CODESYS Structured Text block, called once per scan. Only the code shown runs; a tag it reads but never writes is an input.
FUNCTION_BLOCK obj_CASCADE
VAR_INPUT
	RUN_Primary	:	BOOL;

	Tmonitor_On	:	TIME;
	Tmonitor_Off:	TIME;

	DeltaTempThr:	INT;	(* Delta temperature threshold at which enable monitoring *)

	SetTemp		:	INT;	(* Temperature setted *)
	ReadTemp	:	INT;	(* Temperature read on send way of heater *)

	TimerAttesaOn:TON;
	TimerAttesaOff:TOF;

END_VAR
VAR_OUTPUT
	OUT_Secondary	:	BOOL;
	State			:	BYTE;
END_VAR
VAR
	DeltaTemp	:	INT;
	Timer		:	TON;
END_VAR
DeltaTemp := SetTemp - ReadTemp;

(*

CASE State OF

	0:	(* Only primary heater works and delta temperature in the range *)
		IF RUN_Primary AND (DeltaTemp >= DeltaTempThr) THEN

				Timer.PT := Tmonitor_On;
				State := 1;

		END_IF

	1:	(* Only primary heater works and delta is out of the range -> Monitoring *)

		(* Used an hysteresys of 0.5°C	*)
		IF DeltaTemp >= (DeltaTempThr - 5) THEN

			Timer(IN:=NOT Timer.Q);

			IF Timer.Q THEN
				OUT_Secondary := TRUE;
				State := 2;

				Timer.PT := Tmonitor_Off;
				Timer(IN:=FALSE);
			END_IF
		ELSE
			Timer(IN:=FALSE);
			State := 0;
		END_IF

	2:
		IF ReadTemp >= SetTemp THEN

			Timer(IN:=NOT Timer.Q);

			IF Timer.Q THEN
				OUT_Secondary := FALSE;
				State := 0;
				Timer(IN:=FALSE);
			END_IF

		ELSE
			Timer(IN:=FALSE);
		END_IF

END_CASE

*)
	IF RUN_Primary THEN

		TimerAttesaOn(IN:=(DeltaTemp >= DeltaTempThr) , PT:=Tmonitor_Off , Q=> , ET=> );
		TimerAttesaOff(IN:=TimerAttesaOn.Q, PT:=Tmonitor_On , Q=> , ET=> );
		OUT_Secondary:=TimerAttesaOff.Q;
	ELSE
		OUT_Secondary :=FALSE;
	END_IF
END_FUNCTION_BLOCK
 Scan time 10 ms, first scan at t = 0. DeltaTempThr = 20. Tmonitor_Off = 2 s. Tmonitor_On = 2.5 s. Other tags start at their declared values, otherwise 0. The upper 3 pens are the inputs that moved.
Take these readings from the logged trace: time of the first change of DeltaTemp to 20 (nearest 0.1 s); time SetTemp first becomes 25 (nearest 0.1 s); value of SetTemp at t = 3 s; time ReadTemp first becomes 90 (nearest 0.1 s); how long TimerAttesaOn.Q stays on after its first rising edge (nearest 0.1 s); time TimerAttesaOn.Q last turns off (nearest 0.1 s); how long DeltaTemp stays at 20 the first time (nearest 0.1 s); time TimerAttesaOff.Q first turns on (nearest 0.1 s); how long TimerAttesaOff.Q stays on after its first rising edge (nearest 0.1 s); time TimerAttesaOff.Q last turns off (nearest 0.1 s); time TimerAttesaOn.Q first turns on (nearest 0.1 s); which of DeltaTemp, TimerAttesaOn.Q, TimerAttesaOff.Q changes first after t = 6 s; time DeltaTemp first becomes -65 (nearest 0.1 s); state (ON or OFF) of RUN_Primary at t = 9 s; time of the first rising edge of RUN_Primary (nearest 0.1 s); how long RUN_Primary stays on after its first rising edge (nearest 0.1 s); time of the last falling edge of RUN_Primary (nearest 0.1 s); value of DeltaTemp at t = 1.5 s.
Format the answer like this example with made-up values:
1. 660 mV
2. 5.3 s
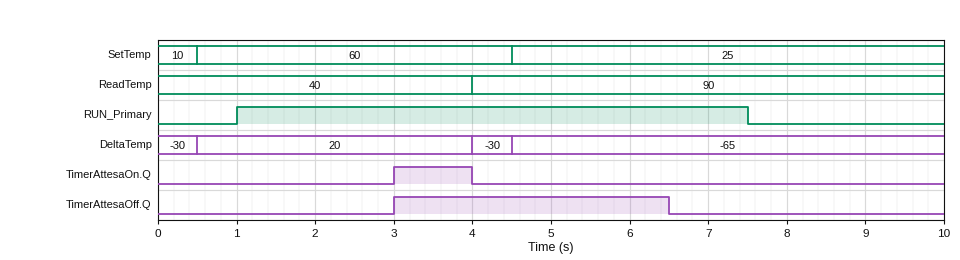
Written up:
1. 0.5 s
2. 4.5 s
3. 60
4. 4.0 s
5. 1.0 s
6. 4.0 s
7. 3.5 s
8. 3.0 s
9. 3.5 s
10. 6.5 s
11. 3.0 s
12. TimerAttesaOff.Q
13. 4.5 s
14. OFF
15. 1.0 s
16. 6.5 s
17. 7.5 s
18. 20
